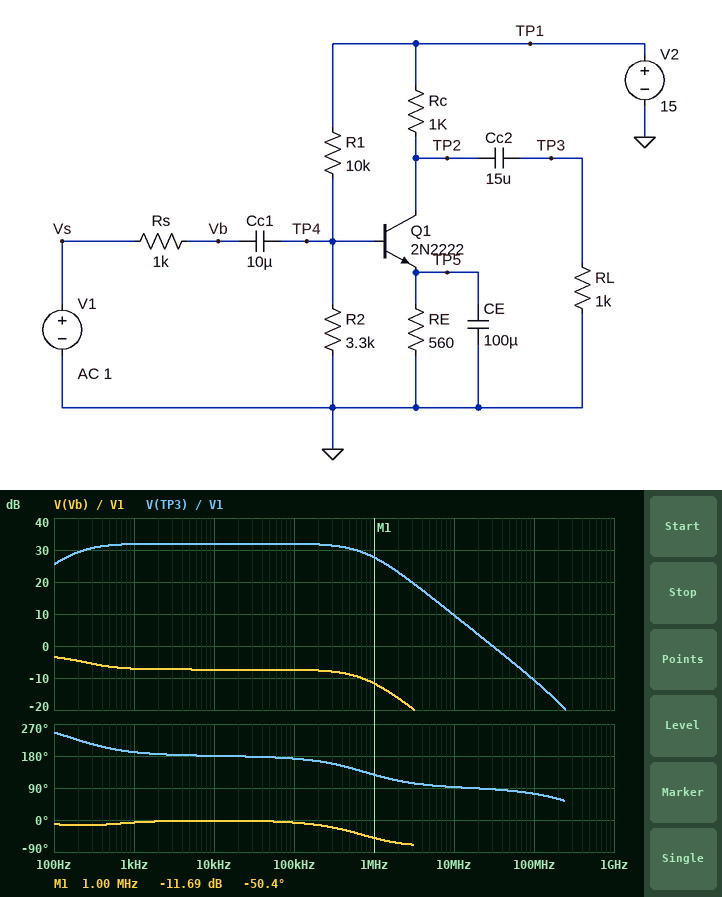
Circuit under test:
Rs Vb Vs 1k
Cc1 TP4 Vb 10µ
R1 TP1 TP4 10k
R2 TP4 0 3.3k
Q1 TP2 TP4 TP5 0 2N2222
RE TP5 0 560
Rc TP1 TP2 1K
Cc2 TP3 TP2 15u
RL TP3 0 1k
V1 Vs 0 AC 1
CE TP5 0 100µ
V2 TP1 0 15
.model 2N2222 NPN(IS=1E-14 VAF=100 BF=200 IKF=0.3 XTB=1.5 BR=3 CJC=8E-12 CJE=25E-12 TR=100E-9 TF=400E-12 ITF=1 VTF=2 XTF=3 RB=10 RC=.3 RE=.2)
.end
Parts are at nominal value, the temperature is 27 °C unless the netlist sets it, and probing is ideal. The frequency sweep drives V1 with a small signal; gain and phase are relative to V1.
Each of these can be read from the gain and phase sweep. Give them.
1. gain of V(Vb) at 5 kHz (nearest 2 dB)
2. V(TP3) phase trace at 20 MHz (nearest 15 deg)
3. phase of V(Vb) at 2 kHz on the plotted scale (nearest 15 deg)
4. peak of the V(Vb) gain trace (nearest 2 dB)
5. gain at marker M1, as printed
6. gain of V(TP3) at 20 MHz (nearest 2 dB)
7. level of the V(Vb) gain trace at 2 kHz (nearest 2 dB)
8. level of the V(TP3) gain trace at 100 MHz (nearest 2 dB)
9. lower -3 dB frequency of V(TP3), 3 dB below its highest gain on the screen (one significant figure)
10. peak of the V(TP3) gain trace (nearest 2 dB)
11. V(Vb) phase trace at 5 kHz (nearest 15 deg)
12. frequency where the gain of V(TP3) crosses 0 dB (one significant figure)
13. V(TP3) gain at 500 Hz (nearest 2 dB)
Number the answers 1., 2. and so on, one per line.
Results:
1. -8 dB
2. 90 deg
3. 0 deg
4. -4 dB
5. -11.69 dB
6. 4 dB
7. -8 dB
8. -10 dB
9. 200 Hz
10. 32 dB
11. 0 deg
12. 30 MHz
13. 32 dB
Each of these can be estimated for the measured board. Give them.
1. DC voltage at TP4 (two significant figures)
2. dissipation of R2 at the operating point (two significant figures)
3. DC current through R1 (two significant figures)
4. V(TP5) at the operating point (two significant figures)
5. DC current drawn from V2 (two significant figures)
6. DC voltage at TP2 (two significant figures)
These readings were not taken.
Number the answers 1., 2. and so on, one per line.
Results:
1. 3.7 V
2. 4.1 mW
3. 1.1 mA
4. 3.0 V
5. 6.4 mA
6. 9.7 V
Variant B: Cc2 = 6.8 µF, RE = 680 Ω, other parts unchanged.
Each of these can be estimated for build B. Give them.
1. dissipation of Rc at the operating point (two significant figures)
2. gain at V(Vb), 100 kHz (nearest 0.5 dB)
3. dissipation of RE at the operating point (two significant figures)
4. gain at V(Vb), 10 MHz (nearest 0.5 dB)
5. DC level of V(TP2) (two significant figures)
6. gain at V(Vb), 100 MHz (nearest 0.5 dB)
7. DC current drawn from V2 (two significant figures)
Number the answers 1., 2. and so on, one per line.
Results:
1. 19 mW
2. -7.0 dB
3. 13 mW
4. -27.5 dB
5. 11 V
6. -37.0 dB
7. 5.5 mA
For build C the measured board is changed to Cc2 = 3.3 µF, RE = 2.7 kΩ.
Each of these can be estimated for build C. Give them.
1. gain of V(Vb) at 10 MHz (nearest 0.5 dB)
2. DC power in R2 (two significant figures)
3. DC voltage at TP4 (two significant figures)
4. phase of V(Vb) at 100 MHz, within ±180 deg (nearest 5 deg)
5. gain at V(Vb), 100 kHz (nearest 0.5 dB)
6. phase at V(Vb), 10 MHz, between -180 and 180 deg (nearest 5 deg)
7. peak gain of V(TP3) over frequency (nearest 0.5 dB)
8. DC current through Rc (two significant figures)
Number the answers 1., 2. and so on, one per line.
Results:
1. -18.5 dB
2. 4.2 mW
3. 3.7 V
4. -40 deg
5. -4.0 dB
6. -70 deg
7. 22.5 dB
8. 1.1 mA
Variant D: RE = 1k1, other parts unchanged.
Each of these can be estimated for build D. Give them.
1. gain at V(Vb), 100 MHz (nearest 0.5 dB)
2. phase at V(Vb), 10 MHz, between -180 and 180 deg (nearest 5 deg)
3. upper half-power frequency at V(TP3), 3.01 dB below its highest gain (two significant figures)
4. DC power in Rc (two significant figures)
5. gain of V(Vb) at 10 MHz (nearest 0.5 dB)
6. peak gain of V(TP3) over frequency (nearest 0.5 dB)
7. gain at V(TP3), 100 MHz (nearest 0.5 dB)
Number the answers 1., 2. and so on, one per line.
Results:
1. -36.0 dB
2. -70 deg
3. 1.1 MHz
4. 7.4 mW
5. -24.0 dB
6. 28.5 dB
7. -11.0 dB
